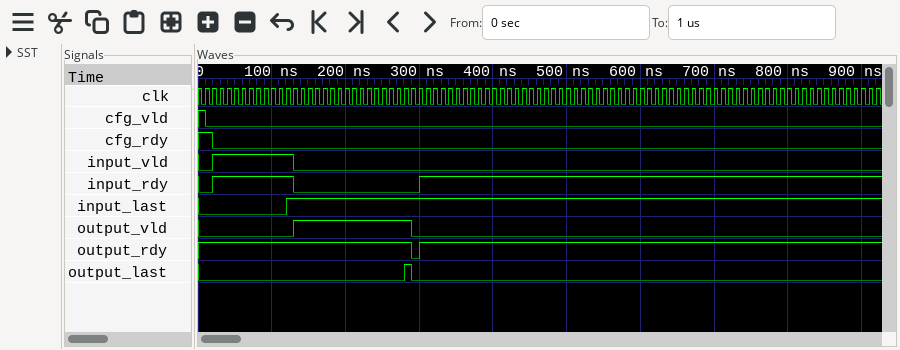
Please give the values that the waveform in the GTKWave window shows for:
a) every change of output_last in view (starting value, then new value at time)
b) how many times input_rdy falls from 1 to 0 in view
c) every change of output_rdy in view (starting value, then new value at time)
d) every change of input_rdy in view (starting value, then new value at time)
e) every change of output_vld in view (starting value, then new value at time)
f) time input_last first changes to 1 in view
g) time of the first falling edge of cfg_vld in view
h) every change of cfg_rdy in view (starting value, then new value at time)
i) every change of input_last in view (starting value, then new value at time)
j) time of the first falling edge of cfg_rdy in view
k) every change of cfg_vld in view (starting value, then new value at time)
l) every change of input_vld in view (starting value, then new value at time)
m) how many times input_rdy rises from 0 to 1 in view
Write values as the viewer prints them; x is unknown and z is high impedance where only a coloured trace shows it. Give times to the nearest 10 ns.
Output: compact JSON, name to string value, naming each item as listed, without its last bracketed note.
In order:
{"every change of output_last in view": "0, 1 at 280 ns, 0 at 290 ns", "how many times input_rdy falls from 1 to 0 in view": "1", "every change of output_rdy in view": "1, 0 at 290 ns, 1 at 300 ns", "every change of input_rdy in view": "0, 1 at 20 ns, 0 at 130 ns, 1 at 300 ns", "every change of output_vld in view": "0, 1 at 130 ns, 0 at 290 ns", "time input_last first changes to 1 in view": "120 ns", "time of the first falling edge of cfg_vld in view": "10 ns", "every change of cfg_rdy in view": "1, 0 at 20 ns", "every change of input_last in view": "0, 1 at 120 ns", "time of the first falling edge of cfg_rdy in view": "20 ns", "every change of cfg_vld in view": "1, 0 at 10 ns", "every change of input_vld in view": "0, 1 at 20 ns, 0 at 130 ns", "how many times input_rdy rises from 0 to 1 in view": "2"}
